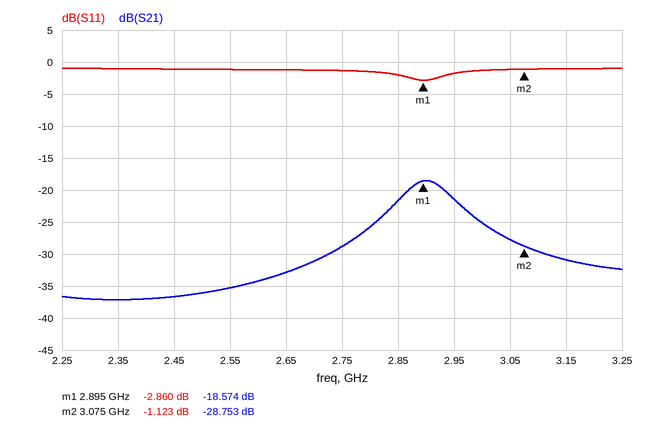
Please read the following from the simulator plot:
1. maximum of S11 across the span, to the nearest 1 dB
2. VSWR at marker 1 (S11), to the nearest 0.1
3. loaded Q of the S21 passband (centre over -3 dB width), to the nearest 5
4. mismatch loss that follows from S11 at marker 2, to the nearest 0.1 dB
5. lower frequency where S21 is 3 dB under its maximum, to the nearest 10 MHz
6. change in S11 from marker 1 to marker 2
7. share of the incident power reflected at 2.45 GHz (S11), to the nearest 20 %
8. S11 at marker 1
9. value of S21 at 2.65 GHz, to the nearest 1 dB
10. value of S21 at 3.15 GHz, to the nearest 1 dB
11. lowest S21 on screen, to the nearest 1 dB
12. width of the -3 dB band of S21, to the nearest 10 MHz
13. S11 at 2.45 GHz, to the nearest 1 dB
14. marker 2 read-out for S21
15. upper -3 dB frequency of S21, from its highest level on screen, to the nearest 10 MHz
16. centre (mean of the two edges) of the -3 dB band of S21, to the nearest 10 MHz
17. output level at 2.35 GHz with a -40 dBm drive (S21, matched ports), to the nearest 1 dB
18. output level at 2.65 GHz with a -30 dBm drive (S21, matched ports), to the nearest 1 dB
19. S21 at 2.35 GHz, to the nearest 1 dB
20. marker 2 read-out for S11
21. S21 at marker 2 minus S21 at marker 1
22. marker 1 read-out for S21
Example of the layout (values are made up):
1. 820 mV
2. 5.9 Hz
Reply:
1. -1 dB
2. 6.1
3. 30
4. 6.4 dB
5. 2.85 GHz
6. 1.737 dB
7. 80 %
8. -2.860 dB
9. -33 dB
10. -31 dB
11. -37 dB
12. 100 MHz
13. -1 dB
14. -28.753 dB
15. 2.95 GHz
16. 2.90 GHz
17. -77 dBm
18. -63 dBm
19. -37 dB
20. -1.123 dB
21. -10.179 dB
22. -18.574 dB
